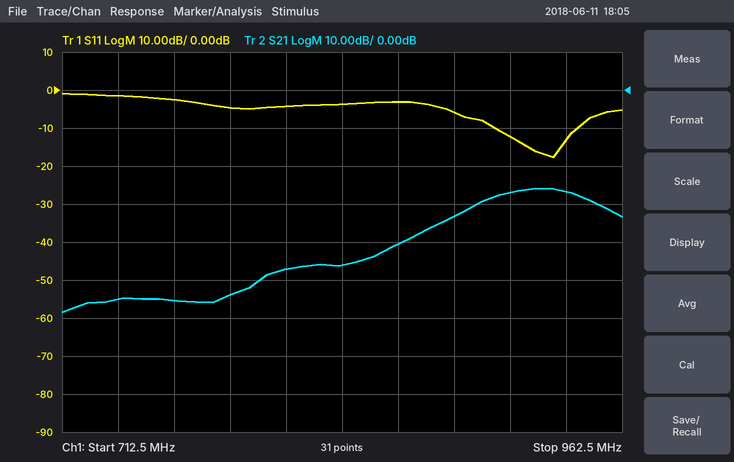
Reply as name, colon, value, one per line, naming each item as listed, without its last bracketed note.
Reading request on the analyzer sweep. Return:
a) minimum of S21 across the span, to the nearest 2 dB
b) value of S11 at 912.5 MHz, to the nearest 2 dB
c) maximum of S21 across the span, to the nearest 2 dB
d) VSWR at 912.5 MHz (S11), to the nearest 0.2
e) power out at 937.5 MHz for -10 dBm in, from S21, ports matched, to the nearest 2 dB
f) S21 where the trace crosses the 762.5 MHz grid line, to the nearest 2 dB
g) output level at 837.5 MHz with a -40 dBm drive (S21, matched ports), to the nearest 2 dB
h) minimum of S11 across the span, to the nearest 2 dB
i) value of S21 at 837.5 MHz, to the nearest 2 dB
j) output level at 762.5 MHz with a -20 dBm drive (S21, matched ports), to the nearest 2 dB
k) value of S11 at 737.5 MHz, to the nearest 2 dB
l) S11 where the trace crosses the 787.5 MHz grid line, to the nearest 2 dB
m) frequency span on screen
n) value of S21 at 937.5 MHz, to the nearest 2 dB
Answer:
minimum of S21 across the span, to the nearest 2 dB: -58 dB
value of S11 at 912.5 MHz, to the nearest 2 dB: -12 dB
maximum of S21 across the span, to the nearest 2 dB: -26 dB
VSWR at 912.5 MHz (S11), to the nearest 0.2: 1.6
power out at 937.5 MHz for -10 dBm in, from S21, ports matched, to the nearest 2 dB: -36 dBm
S21 where the trace crosses the 762.5 MHz grid line, to the nearest 2 dB: -56 dB
output level at 837.5 MHz with a -40 dBm drive (S21, matched ports), to the nearest 2 dB: -86 dBm
minimum of S11 across the span, to the nearest 2 dB: -18 dB
value of S21 at 837.5 MHz, to the nearest 2 dB: -46 dB
output level at 762.5 MHz with a -20 dBm drive (S21, matched ports), to the nearest 2 dB: -76 dBm
value of S11 at 737.5 MHz, to the nearest 2 dB: -2 dB
S11 where the trace crosses the 787.5 MHz grid line, to the nearest 2 dB: -4 dB
frequency span on screen: 250 MHz
value of S21 at 937.5 MHz, to the nearest 2 dB: -26 dB
